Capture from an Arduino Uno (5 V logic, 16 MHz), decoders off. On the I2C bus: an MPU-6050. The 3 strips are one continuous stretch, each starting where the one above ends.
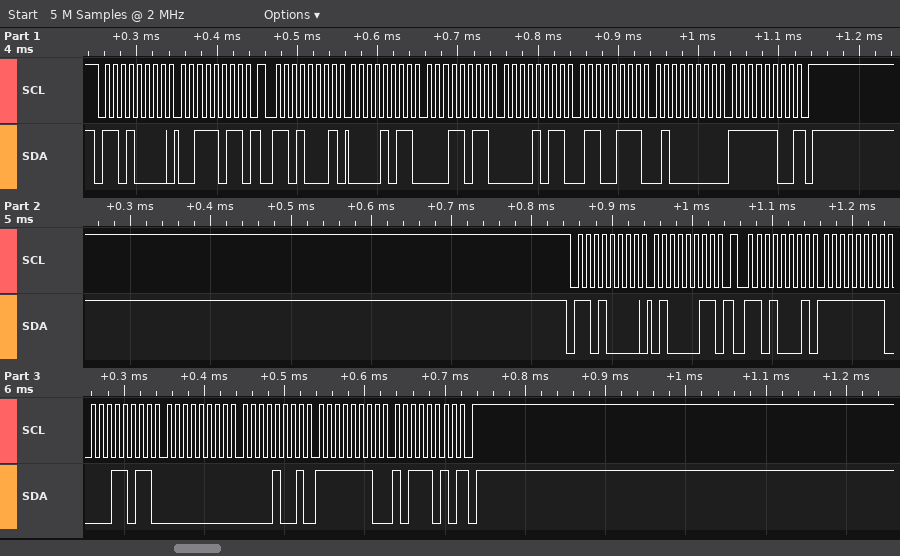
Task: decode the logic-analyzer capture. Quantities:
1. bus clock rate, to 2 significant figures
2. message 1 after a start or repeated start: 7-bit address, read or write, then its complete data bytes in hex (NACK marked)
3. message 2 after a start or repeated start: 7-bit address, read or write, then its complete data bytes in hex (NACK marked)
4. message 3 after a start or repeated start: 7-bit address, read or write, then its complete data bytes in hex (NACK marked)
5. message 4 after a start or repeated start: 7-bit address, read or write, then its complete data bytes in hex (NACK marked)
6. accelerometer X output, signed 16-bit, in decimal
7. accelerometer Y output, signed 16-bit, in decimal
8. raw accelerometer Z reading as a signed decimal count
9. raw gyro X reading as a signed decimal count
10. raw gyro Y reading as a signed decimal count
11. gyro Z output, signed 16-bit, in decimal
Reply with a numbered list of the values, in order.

1. 100 kHz
2. 0x68 write: 3B
3. 0x68 read: 0B 1B 0B 67 40 FC NACK
4. 0x68 write: 43
5. 0x68 read: FF 1B 00 09 FE BA NACK
6. 2843
7. 2919
8. 16636
9. -229
10. 9
11. -326
